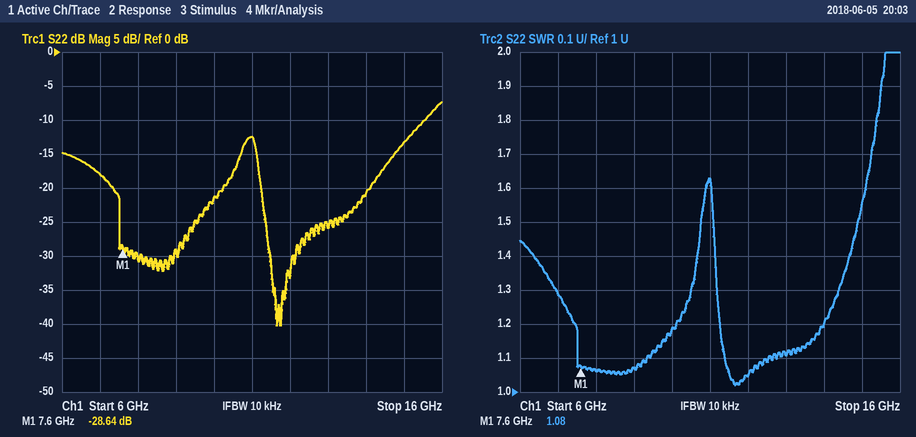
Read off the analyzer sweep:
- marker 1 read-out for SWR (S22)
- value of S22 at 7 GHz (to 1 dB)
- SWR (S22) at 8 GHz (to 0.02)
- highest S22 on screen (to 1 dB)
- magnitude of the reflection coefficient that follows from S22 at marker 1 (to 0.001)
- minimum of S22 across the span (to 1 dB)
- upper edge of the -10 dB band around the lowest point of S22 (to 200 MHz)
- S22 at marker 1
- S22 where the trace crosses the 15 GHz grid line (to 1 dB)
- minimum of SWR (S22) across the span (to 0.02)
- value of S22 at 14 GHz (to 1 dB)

1.08
-18 dB
1.06
-7 dB
0.037
-40 dB
15.6 GHz
-28.64 dB
-13 dB
1.02
-21 dB
